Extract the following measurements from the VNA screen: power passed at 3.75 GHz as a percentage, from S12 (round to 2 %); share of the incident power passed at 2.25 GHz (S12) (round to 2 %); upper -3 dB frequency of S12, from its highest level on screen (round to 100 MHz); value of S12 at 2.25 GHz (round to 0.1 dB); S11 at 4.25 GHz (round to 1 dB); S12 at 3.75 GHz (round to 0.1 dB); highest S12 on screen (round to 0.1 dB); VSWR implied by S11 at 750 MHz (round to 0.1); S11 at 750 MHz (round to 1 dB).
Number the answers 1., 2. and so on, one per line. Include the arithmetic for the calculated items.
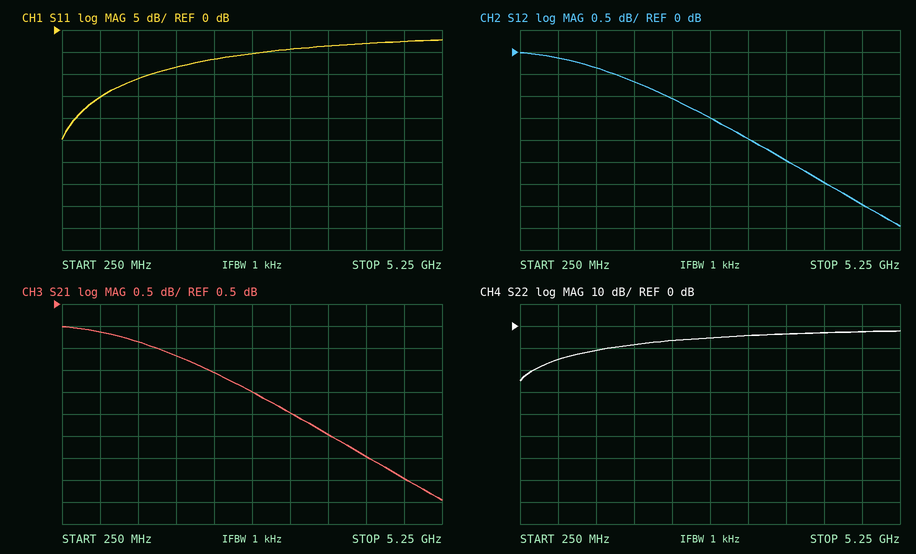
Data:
1. 10^(-2.5/10) ≈ 56 %
2. 10^(-1.1/10) ≈ 78 %
3. 4.3 GHz
4. -1.1 dB
5. -3 dB
6. -2.5 dB
7. 0.0 dB
8. |Γ| = 10^(-15/20) = 0.1778; VSWR = (1 + 0.1778)/(1 − 0.1778) ≈ 1.4
9. -15 dB
